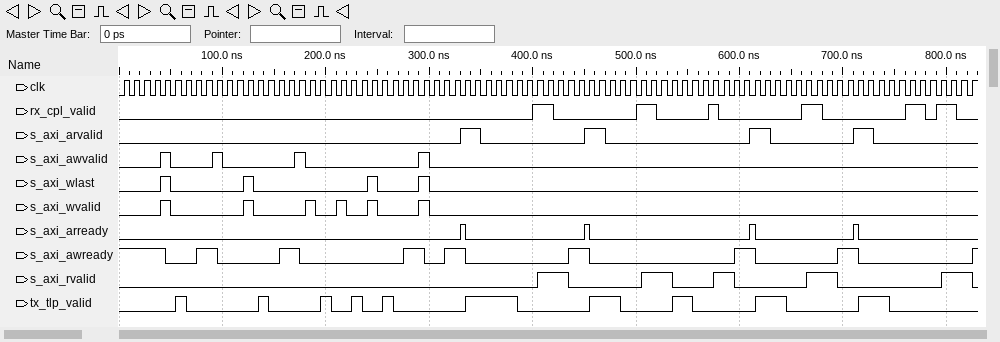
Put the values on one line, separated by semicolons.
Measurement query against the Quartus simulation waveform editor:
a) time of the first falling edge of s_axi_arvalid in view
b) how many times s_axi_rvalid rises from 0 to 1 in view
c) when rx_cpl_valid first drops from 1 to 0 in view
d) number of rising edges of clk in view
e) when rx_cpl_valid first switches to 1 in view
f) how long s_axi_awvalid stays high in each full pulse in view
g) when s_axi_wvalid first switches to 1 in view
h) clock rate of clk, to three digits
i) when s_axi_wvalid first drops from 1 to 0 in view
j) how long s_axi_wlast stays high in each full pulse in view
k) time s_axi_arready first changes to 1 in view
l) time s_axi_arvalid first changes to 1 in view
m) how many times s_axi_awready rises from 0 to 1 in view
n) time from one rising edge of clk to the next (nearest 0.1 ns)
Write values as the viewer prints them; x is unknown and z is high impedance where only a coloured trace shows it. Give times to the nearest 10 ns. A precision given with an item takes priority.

350 ns; 5; 420 ns; 83; 400 ns; 10 ns, 10 ns, 10 ns, 10 ns; 40 ns; 100 MHz; 50 ns; 10 ns, 10 ns, 10 ns, 10 ns; 330 ns; 330 ns; 8; 10 ns
